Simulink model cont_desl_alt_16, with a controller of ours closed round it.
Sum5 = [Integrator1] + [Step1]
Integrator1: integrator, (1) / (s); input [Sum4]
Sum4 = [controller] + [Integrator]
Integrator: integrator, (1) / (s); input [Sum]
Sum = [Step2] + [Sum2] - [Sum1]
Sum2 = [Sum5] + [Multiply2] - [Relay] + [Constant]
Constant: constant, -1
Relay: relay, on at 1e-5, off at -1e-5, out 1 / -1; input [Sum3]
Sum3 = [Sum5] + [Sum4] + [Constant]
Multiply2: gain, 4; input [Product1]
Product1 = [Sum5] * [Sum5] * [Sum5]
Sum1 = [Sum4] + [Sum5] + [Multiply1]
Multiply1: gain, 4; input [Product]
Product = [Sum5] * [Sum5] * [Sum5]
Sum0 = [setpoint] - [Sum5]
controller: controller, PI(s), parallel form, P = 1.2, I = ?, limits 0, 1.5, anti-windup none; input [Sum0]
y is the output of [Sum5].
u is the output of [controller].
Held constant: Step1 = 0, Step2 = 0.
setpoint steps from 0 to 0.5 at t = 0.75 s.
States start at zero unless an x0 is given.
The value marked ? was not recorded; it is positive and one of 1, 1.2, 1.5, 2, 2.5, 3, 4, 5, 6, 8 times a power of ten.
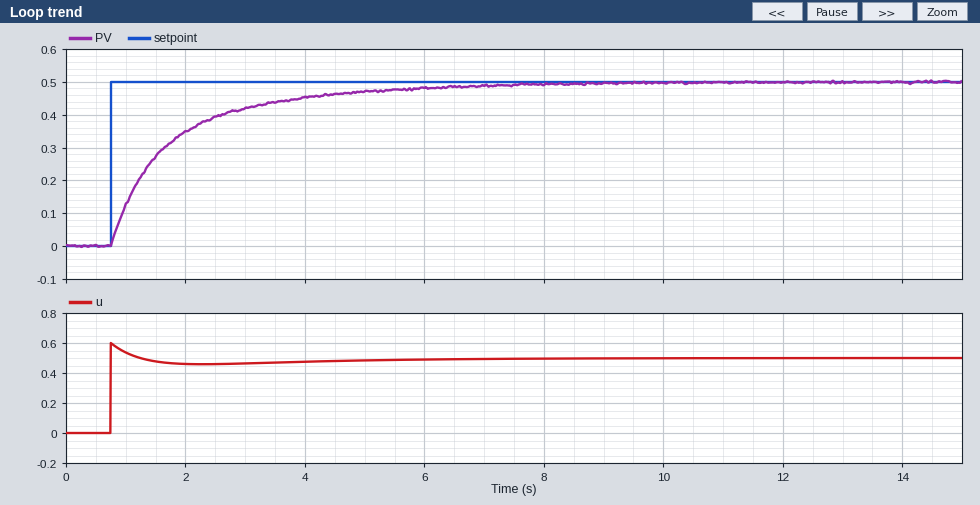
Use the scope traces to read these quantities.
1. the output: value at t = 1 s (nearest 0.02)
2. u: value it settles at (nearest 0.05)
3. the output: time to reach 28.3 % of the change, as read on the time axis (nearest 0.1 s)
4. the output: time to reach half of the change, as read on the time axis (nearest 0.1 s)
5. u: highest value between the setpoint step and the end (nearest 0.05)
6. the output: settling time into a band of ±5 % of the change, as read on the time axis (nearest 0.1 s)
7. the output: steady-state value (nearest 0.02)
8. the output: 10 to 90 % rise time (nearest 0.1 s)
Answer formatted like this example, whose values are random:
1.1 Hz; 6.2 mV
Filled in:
0.12; 0.50; 1.0 s; 1.4 s; 0.60; 5.4 s; 0.50; 3.1 s
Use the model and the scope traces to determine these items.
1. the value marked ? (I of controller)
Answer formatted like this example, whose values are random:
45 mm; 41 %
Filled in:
0.8
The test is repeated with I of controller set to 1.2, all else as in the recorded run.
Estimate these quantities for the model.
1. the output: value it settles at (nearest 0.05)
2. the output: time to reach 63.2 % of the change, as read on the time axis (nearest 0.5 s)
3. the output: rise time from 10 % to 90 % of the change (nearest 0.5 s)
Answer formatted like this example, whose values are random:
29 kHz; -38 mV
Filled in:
0.50; 1.5 s; 2.0 s
